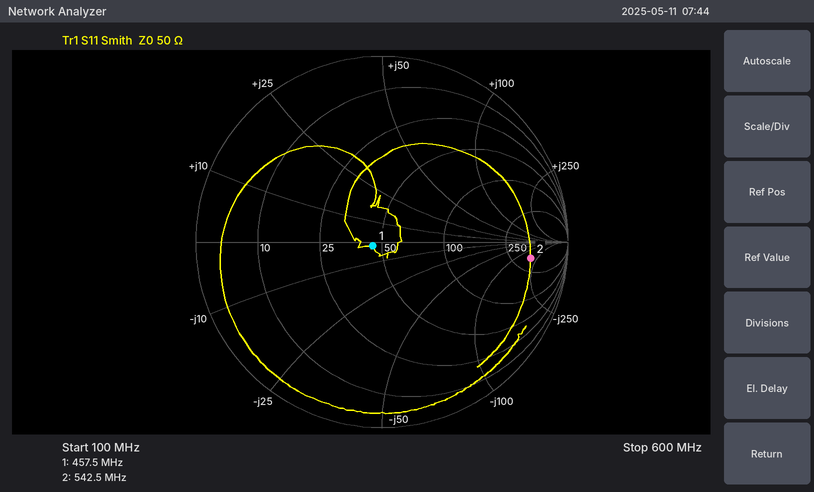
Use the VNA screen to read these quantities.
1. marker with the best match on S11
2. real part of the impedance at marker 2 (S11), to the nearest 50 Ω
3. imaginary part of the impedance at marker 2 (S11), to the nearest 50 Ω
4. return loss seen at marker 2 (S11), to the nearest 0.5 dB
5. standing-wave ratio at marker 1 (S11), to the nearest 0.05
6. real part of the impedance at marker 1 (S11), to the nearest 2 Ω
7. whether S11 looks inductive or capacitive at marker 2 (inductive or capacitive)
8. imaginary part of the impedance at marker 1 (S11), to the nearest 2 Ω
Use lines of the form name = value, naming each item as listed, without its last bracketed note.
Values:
marker with the best match on S11 = marker 1
real part of the impedance at marker 2 (S11), to the nearest 50 Ω = 350 Ω
imaginary part of the impedance at marker 2 (S11), to the nearest 50 Ω = -200 Ω
return loss seen at marker 2 (S11), to the nearest 0.5 dB = 2.0 dB
standing-wave ratio at marker 1 (S11), to the nearest 0.05 = 1.10
real part of the impedance at marker 1 (S11), to the nearest 2 Ω = 46 Ω
whether S11 looks inductive or capacitive at marker 2 = capacitive
imaginary part of the impedance at marker 1 (S11), to the nearest 2 Ω = -2 Ω
